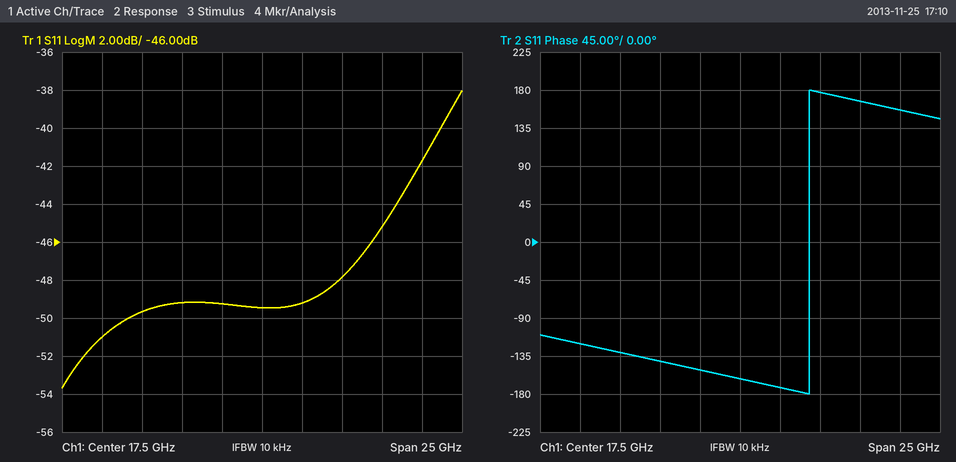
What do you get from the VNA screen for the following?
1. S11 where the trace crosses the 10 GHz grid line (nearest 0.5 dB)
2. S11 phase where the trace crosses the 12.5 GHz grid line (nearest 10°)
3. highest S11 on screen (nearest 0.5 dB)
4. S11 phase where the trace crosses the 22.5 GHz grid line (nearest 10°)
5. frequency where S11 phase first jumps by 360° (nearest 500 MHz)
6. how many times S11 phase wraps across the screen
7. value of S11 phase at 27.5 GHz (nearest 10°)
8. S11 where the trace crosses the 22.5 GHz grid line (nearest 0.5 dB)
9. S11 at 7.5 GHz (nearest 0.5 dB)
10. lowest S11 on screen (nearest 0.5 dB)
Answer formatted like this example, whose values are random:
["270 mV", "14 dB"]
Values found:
["-49.5 dB", "-140°", "-38.0 dB", "180°", "22.0 GHz", "1", "160°", "-48.0 dB", "-51.0 dB", "-53.5 dB"]
